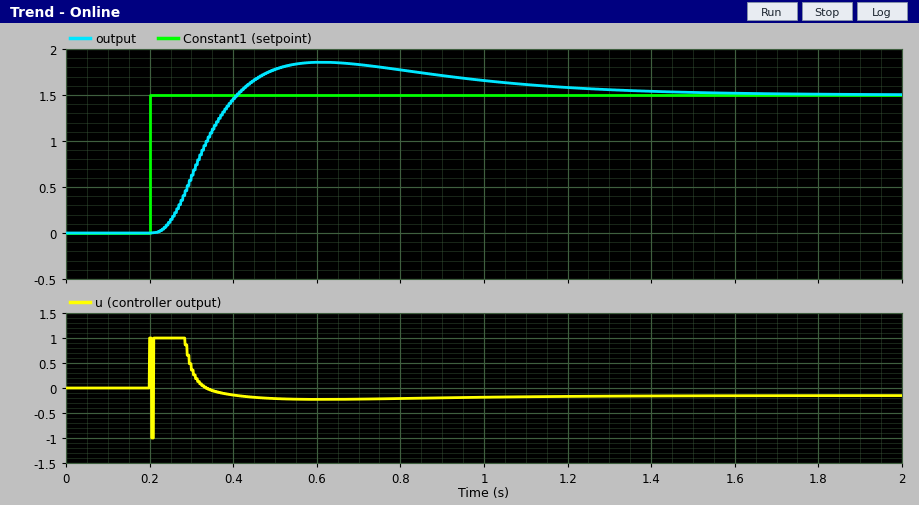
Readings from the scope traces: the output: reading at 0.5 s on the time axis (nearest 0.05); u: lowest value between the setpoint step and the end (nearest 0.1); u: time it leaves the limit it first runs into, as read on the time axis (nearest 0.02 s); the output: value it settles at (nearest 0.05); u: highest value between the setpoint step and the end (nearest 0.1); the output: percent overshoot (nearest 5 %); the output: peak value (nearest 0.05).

1.80
-1.0
0.28 s
1.50
1.0
25 %
1.85
